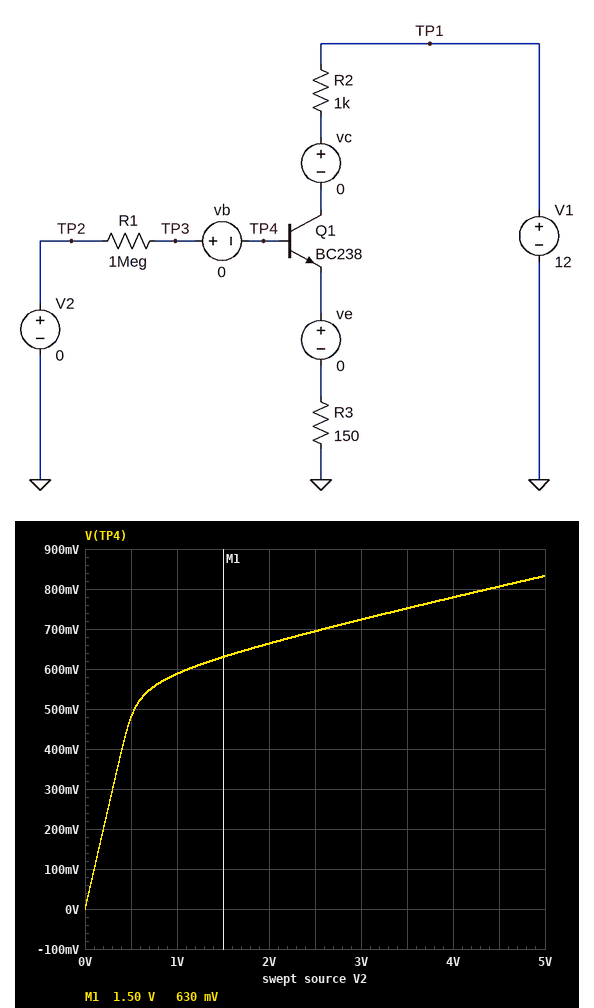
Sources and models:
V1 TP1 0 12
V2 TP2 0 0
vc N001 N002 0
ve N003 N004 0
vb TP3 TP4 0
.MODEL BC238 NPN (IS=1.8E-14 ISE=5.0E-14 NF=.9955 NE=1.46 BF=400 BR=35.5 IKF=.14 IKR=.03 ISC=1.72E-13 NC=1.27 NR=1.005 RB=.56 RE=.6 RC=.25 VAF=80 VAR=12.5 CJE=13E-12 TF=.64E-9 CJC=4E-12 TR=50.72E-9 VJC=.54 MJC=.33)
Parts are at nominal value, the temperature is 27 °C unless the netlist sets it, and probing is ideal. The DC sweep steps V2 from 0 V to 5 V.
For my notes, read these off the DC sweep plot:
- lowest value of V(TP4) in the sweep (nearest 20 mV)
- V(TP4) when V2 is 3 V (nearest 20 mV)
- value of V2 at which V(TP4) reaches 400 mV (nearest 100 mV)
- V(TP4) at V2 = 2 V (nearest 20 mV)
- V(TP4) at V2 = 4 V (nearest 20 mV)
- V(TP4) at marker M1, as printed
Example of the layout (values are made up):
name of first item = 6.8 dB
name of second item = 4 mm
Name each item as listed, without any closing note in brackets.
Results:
lowest value of V(TP4) in the sweep = 0 V
V(TP4) when V2 is 3 V = 720 mV
value of V2 at which V(TP4) reaches 400 mV = 400 mV
V(TP4) at V2 = 2 V = 660 mV
V(TP4) at V2 = 4 V = 780 mV
V(TP4) at marker M1, as printed = 630 mV
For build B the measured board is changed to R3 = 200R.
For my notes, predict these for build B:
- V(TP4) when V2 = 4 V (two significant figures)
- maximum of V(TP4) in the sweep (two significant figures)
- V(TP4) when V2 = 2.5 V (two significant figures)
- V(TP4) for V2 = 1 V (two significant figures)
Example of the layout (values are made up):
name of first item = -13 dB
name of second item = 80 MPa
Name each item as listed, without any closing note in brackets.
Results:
V(TP4) when V2 = 4 V = 820 mV
maximum of V(TP4) in the sweep = 890 mV
V(TP4) when V2 = 2.5 V = 720 mV
V(TP4) for V2 = 1 V = 590 mV
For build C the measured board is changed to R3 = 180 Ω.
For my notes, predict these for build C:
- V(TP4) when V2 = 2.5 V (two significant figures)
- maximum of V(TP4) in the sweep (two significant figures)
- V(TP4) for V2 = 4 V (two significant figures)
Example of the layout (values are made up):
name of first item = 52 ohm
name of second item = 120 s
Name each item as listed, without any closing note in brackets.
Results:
V(TP4) when V2 = 2.5 V = 710 mV
maximum of V(TP4) in the sweep = 870 mV
V(TP4) for V2 = 4 V = 810 mV
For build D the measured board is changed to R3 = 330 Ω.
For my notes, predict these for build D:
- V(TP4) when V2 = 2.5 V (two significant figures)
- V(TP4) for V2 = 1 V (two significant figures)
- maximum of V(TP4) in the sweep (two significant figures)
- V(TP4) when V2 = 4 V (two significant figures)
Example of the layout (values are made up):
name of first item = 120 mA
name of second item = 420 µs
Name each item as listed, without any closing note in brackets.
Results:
V(TP4) when V2 = 2.5 V = 780 mV
V(TP4) for V2 = 1 V = 600 mV
maximum of V(TP4) in the sweep = 1.0 V
V(TP4) when V2 = 4 V = 930 mV
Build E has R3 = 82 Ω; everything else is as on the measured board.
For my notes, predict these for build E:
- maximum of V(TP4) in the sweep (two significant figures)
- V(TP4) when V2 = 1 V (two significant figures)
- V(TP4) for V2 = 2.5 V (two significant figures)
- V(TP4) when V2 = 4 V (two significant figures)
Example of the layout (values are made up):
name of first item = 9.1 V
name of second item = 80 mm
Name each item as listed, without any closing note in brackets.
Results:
maximum of V(TP4) in the sweep = 750 mV
V(TP4) when V2 = 1 V = 580 mV
V(TP4) for V2 = 2.5 V = 660 mV
V(TP4) when V2 = 4 V = 720 mV
